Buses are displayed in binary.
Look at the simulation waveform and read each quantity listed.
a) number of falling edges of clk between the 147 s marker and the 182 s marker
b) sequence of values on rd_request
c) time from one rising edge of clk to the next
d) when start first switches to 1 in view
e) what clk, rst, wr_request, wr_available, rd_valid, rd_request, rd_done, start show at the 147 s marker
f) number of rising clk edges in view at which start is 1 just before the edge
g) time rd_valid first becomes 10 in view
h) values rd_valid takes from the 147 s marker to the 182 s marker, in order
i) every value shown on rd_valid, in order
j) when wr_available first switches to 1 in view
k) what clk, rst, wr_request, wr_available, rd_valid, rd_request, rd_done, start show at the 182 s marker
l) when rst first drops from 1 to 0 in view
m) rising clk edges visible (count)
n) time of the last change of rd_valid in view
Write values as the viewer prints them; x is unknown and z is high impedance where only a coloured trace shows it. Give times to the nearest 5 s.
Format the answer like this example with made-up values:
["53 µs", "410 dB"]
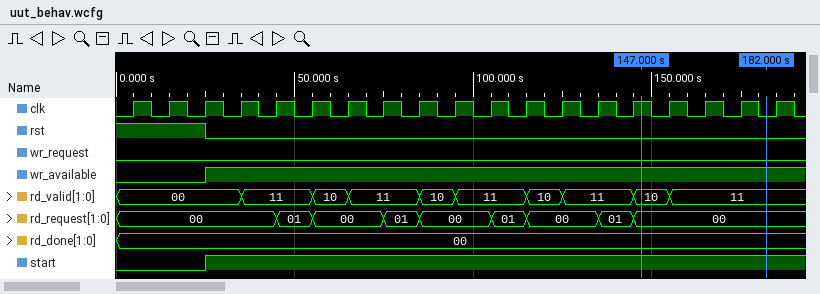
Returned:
["4", "00, 01, 00, 01, 00, 01, 00, 01, 00", "10 s", "25 s", "clk=1, rst=0, wr_request=0, wr_available=1, rd_valid=10, rd_request=00, rd_done=00, start=1", "16", "55 s", "10, 11", "00, 11, 10, 11, 10, 11, 10, 11, 10, 11", "25 s", "clk=0, rst=0, wr_request=0, wr_available=1, rd_valid=11, rd_request=00, rd_done=00, start=1", "25 s", "19", "155 s"]
